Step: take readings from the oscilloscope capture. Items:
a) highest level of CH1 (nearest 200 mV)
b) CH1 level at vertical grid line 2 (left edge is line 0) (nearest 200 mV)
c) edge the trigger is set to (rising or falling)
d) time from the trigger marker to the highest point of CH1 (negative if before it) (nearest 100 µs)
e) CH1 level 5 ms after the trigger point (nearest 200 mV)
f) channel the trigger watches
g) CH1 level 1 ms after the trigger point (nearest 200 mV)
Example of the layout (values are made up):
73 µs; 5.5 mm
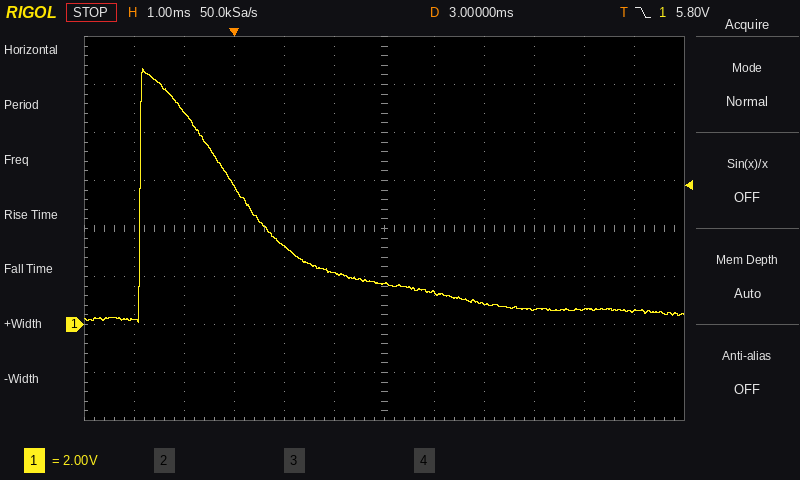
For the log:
10.6 V; 8.8 V; falling; -1.8 ms; 800 mV; CH1; 3.2 V
